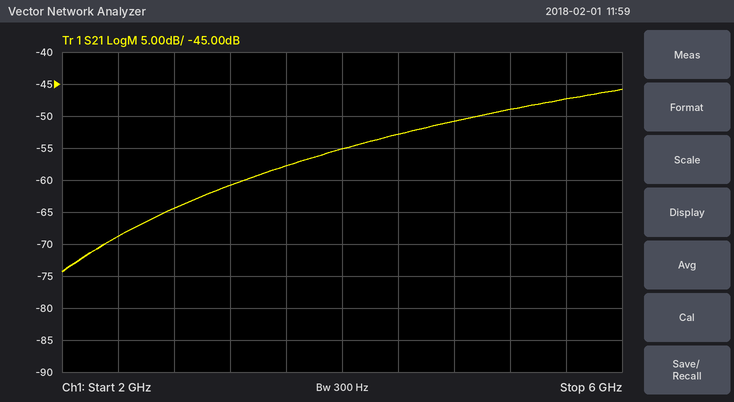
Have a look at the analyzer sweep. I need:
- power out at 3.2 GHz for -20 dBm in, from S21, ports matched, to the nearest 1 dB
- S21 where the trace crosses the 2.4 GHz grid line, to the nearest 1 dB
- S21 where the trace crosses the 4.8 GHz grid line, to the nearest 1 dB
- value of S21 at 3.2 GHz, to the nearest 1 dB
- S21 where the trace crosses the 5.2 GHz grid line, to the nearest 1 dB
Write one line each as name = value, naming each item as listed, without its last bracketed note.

power out at 3.2 GHz for -20 dBm in, from S21, ports matched, to the nearest 1 dB = -81 dBm
S21 where the trace crosses the 2.4 GHz grid line, to the nearest 1 dB = -69 dB
S21 where the trace crosses the 4.8 GHz grid line, to the nearest 1 dB = -51 dB
value of S21 at 3.2 GHz, to the nearest 1 dB = -61 dB
S21 where the trace crosses the 5.2 GHz grid line, to the nearest 1 dB = -49 dB
